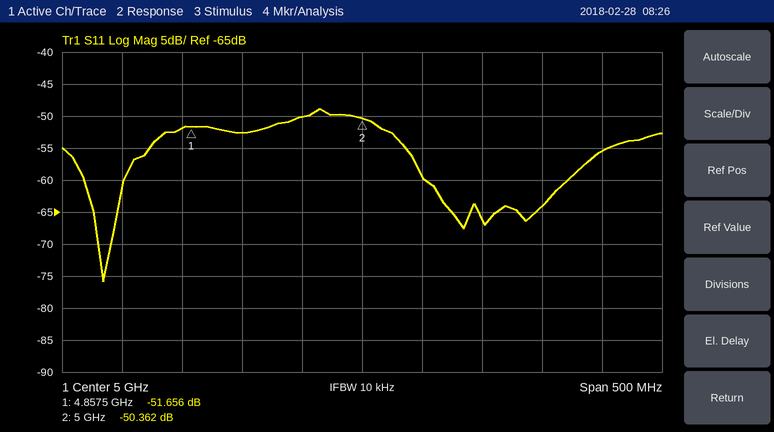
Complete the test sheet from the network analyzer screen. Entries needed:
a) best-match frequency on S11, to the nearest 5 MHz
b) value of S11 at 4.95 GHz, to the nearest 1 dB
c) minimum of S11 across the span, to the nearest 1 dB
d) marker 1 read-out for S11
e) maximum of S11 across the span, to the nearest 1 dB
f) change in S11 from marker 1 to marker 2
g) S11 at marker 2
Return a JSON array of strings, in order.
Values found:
["4.785 GHz", "-50 dB", "-76 dB", "-51.656 dB", "-49 dB", "1.294 dB", "-50.362 dB"]
